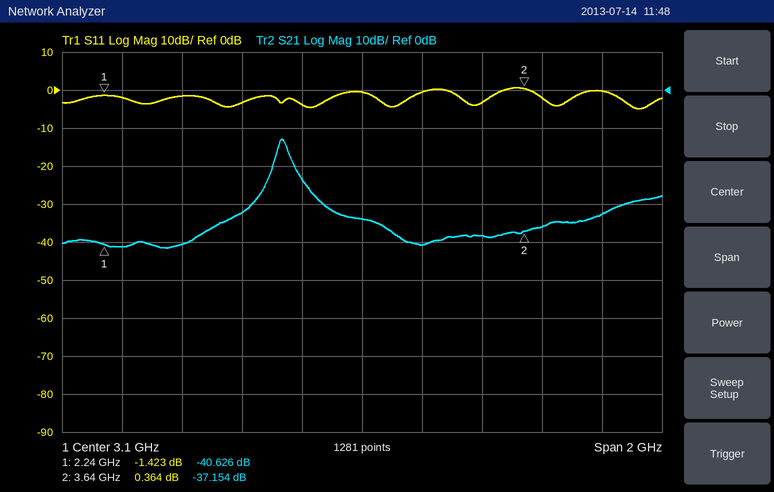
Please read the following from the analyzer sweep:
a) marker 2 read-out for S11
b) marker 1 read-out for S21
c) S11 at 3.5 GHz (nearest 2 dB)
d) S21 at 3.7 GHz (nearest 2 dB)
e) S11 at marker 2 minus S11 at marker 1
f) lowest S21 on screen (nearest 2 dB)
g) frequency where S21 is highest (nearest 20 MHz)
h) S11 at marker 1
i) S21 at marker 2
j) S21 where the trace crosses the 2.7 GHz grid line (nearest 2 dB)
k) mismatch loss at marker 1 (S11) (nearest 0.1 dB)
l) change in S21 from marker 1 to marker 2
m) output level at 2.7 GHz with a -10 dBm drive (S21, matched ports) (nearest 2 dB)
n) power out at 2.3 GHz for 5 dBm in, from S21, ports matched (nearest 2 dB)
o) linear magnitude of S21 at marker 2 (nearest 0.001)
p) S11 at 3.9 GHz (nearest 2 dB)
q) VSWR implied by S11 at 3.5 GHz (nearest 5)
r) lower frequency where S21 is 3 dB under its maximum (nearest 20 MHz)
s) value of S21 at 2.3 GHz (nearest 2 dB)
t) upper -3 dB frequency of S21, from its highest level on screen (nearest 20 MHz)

0.364 dB
-40.626 dB
-4 dB
-36 dB
1.787 dB
-42 dB
2.84 GHz
-1.423 dB
-37.154 dB
-32 dB
5.5 dB
3.472 dB
-42 dBm
-36 dBm
0.014
0 dB
5
2.82 GHz
-42 dB
2.86 GHz
